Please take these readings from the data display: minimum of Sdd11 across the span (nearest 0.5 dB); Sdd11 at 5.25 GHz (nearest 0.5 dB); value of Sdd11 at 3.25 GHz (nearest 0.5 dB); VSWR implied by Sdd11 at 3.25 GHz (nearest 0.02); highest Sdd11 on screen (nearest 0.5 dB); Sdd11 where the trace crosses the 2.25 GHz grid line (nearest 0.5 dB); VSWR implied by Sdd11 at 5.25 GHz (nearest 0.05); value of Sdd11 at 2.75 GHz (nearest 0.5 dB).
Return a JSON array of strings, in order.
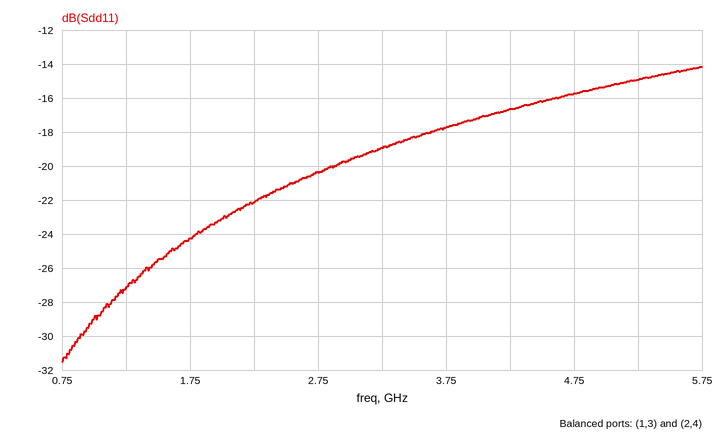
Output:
["-31.5 dB", "-15.0 dB", "-19.0 dB", "1.26", "-14.0 dB", "-22.0 dB", "1.45", "-20.5 dB"]
